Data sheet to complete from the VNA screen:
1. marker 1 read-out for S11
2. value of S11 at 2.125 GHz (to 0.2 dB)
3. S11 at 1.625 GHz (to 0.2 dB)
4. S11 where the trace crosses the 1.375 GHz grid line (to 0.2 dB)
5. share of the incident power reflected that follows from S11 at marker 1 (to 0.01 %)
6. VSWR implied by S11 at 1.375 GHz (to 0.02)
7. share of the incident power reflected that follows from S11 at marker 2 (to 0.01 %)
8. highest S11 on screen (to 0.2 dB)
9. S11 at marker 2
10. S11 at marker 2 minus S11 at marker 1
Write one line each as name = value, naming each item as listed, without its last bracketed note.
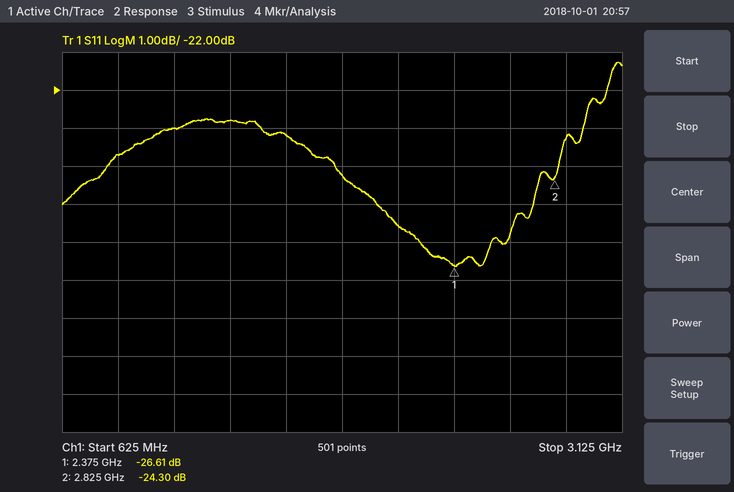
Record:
marker 1 read-out for S11 = -26.61 dB
value of S11 at 2.125 GHz = -25.6 dB
S11 at 1.625 GHz = -23.2 dB
S11 where the trace crosses the 1.375 GHz grid line = -22.8 dB
share of the incident power reflected that follows from S11 at marker 1 = 0.22 %
VSWR implied by S11 at 1.375 GHz = 1.16
share of the incident power reflected that follows from S11 at marker 2 = 0.37 %
highest S11 on screen = -21.2 dB
S11 at marker 2 = -24.30 dB
S11 at marker 2 minus S11 at marker 1 = 2.31 dB
